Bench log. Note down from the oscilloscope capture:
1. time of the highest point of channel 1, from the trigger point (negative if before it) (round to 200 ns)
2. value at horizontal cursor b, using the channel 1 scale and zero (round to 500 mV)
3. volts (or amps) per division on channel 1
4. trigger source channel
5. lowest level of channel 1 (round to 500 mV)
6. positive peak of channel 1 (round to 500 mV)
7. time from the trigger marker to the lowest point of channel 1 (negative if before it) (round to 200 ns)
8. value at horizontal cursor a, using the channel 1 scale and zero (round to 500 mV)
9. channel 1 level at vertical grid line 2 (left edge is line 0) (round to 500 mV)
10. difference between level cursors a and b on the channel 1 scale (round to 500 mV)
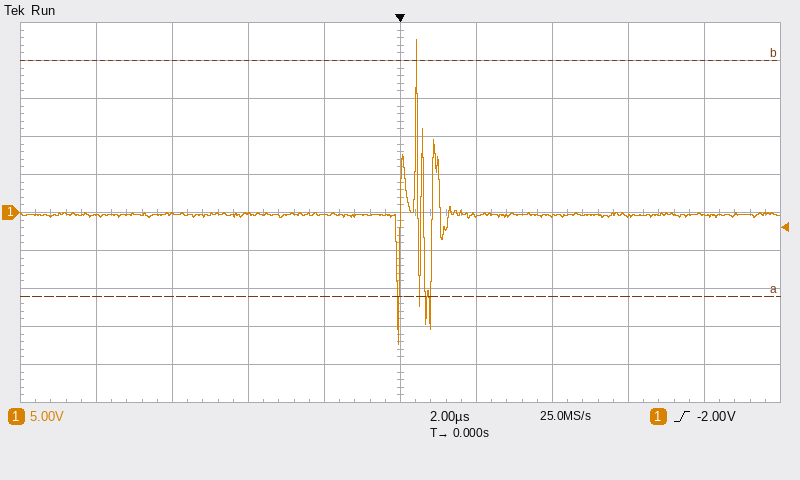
+400 ns
20.0 V
5 V
channel 1
-17.5 V
23.0 V
0.0 µs
-11.0 V
0.0 V
31.0 V
